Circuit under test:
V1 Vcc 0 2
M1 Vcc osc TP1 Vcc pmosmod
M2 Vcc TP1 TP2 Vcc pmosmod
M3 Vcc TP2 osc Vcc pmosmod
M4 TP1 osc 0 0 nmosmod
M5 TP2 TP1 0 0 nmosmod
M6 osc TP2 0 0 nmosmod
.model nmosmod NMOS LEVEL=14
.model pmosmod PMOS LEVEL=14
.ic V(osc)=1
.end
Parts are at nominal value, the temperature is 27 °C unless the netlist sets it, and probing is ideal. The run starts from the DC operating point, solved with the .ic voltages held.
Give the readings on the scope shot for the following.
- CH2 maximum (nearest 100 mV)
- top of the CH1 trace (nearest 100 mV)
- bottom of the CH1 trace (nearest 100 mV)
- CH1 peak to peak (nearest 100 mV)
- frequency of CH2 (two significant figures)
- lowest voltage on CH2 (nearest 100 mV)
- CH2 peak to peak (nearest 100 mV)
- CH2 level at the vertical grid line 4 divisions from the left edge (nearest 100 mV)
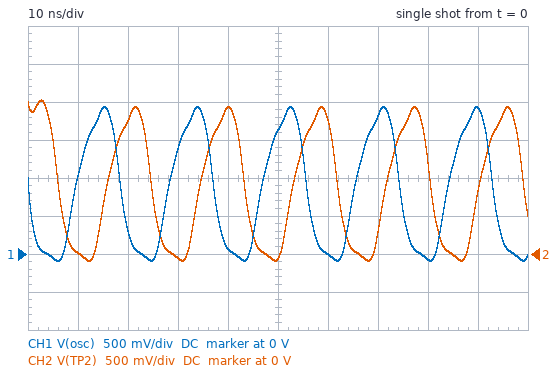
2.0 V
1.9 V
-100 mV
2.0 V
54 MHz
-100 mV
2.1 V
1.9 V
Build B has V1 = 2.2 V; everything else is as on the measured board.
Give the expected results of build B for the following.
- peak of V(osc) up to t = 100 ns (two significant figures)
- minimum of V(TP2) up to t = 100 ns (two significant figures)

2.1 V
-92 mV
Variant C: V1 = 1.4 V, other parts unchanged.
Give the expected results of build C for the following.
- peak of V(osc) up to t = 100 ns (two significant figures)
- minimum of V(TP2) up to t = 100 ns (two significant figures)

1.4 V
-77 mV
